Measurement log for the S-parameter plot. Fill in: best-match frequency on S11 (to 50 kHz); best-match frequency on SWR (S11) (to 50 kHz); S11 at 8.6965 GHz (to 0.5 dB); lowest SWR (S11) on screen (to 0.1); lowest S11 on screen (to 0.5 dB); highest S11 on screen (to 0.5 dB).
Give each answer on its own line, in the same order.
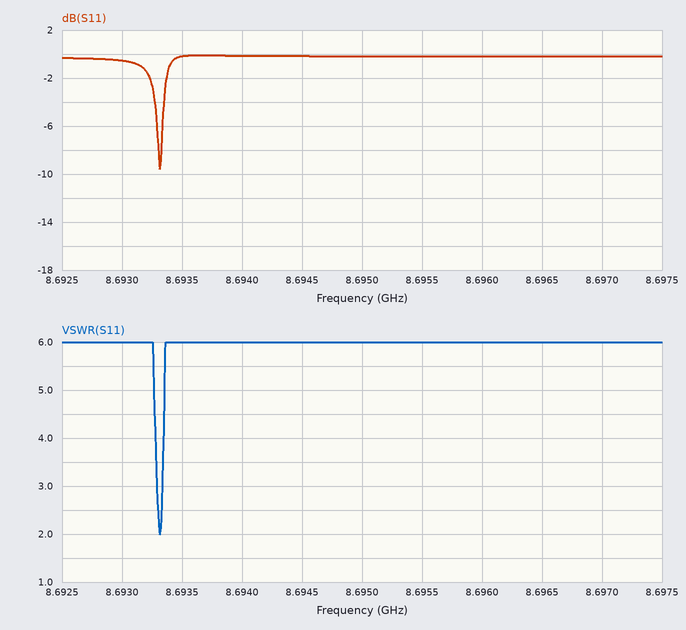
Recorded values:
8.69330 GHz
8.69330 GHz
0.0 dB
2.0
-9.5 dB
0.0 dB
